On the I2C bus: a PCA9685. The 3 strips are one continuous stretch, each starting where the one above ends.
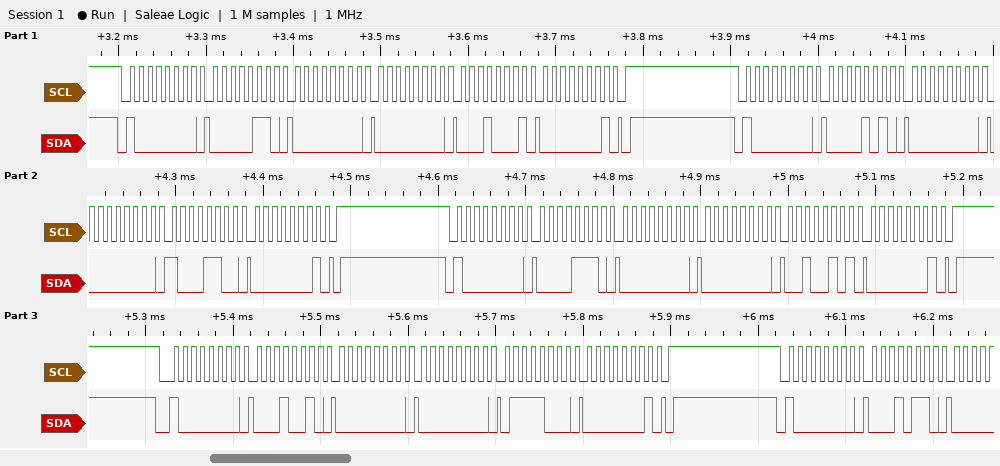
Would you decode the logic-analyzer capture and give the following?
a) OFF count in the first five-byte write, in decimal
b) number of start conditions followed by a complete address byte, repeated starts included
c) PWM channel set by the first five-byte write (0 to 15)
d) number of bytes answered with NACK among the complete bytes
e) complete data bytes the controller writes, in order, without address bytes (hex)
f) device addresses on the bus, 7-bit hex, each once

273
5
0
0
06 00 00 11 01 0A 00 00 8C 01 0E 00 00 25 01 12 00 00 78 01 16
0x40
